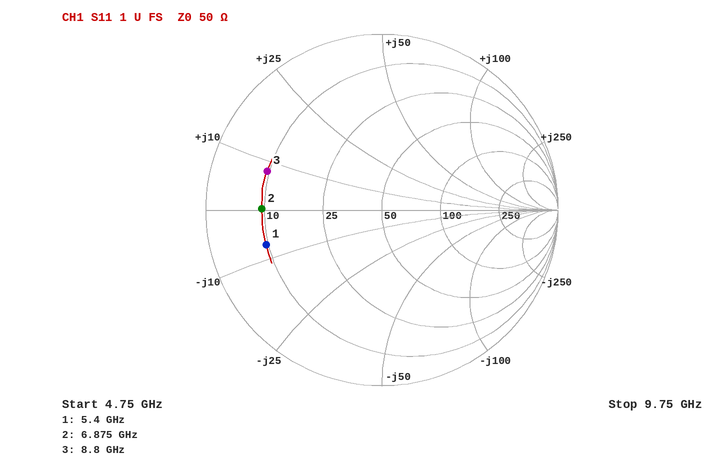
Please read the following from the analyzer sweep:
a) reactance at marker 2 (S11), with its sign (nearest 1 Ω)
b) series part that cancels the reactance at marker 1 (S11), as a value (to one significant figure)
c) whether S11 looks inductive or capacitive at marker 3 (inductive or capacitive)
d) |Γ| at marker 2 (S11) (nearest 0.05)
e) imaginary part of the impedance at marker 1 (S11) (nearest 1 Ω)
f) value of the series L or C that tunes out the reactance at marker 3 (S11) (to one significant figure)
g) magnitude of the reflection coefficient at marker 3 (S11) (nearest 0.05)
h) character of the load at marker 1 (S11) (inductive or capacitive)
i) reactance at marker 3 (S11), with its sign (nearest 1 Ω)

0 Ω
200 pH
inductive
0.70
-7 Ω
2 pF
0.70
capacitive
+8 Ω
